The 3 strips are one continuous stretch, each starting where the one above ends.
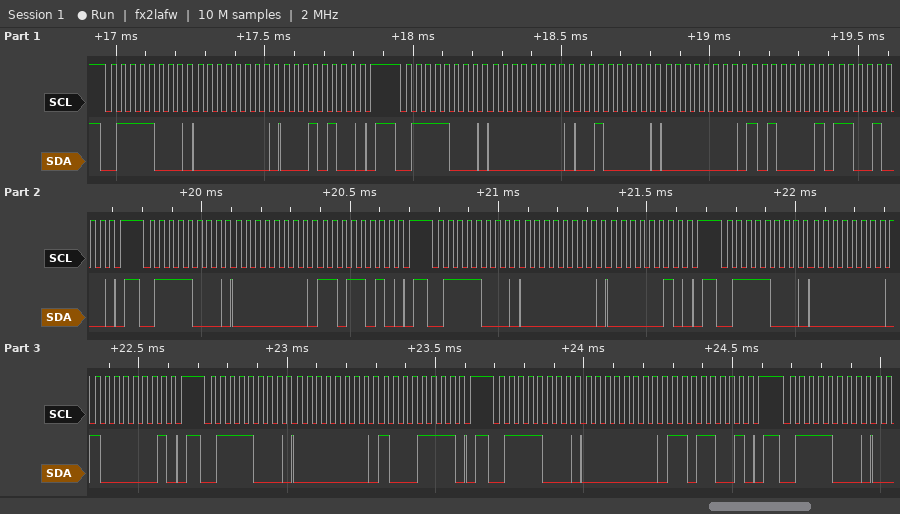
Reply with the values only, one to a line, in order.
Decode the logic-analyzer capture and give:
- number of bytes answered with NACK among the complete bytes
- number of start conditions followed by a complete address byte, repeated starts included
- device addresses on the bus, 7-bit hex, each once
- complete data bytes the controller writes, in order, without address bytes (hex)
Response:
0
8
0x3C
00 14 00 20 00 A1 C8 00 DA 00 02 00 81 00 8F 00 D9
